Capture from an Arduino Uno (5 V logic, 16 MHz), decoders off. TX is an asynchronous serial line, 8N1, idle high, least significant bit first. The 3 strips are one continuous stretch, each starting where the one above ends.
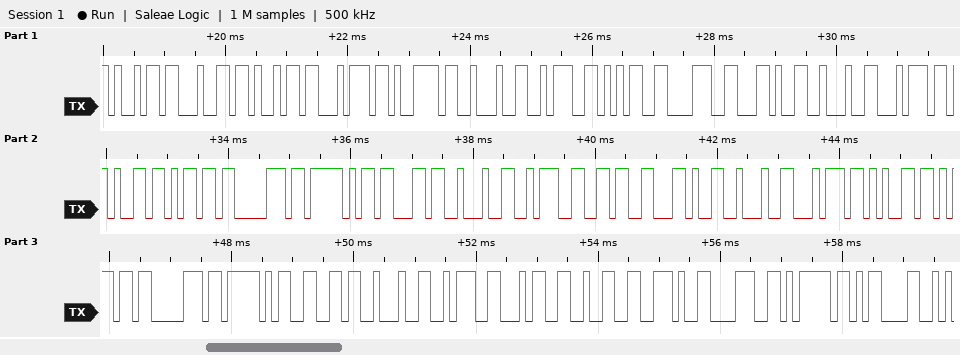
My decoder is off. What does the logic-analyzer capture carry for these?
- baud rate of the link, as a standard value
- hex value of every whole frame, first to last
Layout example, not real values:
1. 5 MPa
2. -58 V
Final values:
1. 9600 baud
2. 69 64 69 74 79 22 3A 35 38 2C 22 74 65 6D 70 5F 63 22 3A 36 2C 22 74 65 6D 70 5F 66 22 3A 34 32 2E 38 7D 0D
